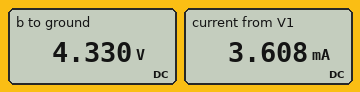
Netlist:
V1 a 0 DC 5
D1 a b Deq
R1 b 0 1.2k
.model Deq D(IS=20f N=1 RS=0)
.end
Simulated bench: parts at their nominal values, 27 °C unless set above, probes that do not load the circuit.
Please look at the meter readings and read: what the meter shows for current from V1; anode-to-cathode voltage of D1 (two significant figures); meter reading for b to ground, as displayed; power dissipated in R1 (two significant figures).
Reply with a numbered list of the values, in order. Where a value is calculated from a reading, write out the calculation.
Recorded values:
1. 3.608 mA
2. 5 V - 4.33 V = 670 mV
3. 4.330 V
4. (4.33 V)^2 / 1.2 kΩ = 16 mW
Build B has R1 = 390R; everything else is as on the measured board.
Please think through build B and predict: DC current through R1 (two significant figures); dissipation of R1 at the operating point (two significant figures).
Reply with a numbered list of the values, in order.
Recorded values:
1. 11 mA
2. 47 mW
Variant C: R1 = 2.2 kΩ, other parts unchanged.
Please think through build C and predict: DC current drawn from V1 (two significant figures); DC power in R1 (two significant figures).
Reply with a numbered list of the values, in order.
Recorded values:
1. 2.0 mA
2. 8.6 mW
